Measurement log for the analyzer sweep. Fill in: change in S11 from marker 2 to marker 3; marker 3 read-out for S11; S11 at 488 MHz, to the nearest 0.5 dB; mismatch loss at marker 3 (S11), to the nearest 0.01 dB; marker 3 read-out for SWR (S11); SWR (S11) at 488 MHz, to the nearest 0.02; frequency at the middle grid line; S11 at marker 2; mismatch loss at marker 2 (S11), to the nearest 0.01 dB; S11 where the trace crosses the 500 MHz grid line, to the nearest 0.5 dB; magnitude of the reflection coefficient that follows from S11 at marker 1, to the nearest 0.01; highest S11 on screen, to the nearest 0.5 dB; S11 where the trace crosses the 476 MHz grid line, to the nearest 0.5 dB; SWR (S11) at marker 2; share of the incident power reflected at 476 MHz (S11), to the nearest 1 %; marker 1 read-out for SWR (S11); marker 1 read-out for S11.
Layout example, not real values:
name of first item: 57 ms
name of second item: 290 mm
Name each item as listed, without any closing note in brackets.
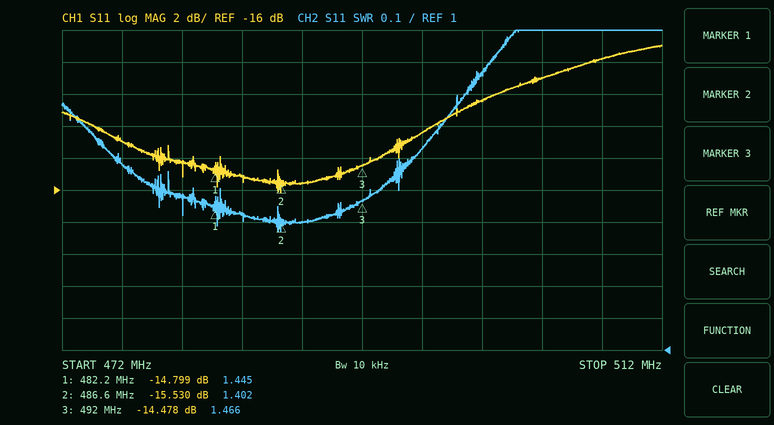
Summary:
change in S11 from marker 2 to marker 3: 1.052 dB
marker 3 read-out for S11: -14.478 dB
S11 at 488 MHz, to the nearest 0.5 dB: -15.5 dB
mismatch loss at marker 3 (S11), to the nearest 0.01 dB: 0.16 dB
marker 3 read-out for SWR: 1.466
SWR (S11) at 488 MHz, to the nearest 0.02: 1.40
frequency at the middle grid line: 492 MHz
S11 at marker 2: -15.530 dB
mismatch loss at marker 2 (S11), to the nearest 0.01 dB: 0.12 dB
S11 where the trace crosses the 500 MHz grid line, to the nearest 0.5 dB: -10.5 dB
magnitude of the reflection coefficient that follows from S11 at marker 1, to the nearest 0.01: 0.18
highest S11 on screen, to the nearest 0.5 dB: -7.0 dB
S11 where the trace crosses the 476 MHz grid line, to the nearest 0.5 dB: -13.0 dB
SWR (S11) at marker 2: 1.402
share of the incident power reflected at 476 MHz (S11), to the nearest 1 %: 5 %
marker 1 read-out for SWR: 1.445
marker 1 read-out for S11: -14.799 dB
